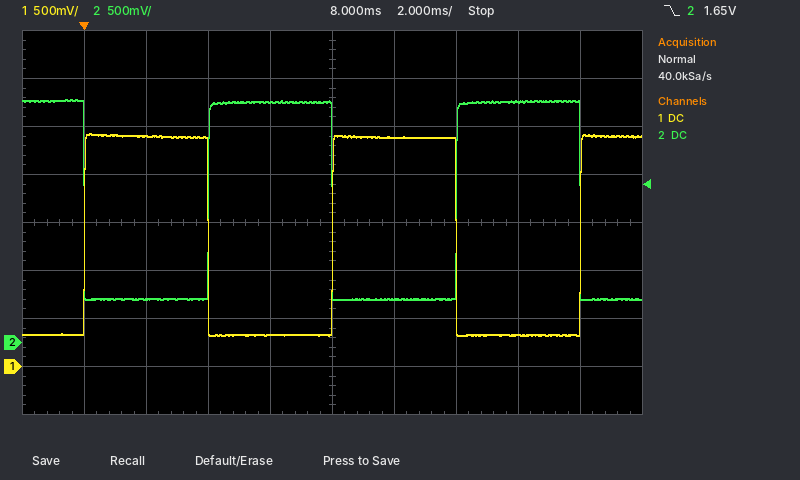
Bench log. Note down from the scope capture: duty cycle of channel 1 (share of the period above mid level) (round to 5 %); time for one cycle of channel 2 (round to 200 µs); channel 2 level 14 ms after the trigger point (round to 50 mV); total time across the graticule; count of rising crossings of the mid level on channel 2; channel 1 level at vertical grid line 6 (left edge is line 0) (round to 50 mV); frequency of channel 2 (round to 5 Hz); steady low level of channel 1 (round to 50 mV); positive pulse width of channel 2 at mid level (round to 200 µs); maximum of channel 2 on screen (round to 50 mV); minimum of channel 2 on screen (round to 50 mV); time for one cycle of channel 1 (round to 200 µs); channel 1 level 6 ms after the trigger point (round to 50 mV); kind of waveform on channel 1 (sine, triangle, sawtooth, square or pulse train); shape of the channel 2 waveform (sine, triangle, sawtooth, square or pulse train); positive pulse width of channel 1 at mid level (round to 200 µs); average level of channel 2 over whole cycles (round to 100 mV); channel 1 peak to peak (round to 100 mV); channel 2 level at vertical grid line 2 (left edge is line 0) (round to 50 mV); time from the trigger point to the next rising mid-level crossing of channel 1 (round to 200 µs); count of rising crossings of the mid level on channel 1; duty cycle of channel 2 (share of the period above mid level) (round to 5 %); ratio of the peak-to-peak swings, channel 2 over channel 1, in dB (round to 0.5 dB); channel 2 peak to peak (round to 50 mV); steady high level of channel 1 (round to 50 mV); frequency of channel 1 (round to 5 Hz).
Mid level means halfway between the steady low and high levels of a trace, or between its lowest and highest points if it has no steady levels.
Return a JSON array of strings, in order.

["50 %", "8.0 ms", "2.50 V", "20 ms", "2", "2.40 V", "125 Hz", "350 mV", "4.0 ms", "2.55 V", "450 mV", "8.0 ms", "350 mV", "square", "square", "4.0 ms", "1.5 V", "2.10 V", "450 mV", "8.0 ms", "3", "50 %", "0.0 dB", "2.10 V", "2.40 V", "125 Hz"]
